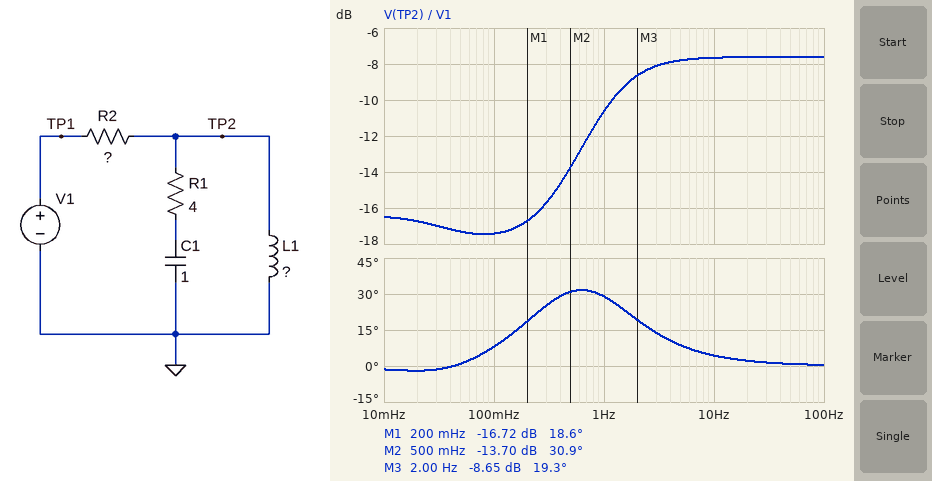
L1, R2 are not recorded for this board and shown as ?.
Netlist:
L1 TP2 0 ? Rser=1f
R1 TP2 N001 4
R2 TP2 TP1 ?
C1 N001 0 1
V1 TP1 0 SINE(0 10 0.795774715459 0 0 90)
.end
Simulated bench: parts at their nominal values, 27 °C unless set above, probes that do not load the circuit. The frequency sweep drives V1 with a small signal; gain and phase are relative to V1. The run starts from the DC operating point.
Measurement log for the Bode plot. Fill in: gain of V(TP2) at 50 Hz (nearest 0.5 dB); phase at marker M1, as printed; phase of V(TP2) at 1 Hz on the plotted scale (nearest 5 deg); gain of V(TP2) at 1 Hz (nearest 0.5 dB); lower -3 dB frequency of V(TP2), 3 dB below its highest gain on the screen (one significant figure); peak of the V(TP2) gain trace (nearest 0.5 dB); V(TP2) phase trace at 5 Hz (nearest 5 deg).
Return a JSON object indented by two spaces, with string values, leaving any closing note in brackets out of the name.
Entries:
{
  "gain of V(TP2) at 50 Hz": "-7.5 dB",
  "phase at marker M1, as printed": "18.6 deg",
  "phase of V(TP2) at 1 Hz on the plotted scale": "30 deg",
  "gain of V(TP2) at 1 Hz": "-10.5 dB",
  "lower -3 dB frequency of V(TP2), 3 dB below its highest gain on the screen": "1 Hz",
  "peak of the V(TP2) gain trace": "-7.5 dB",
  "V(TP2) phase trace at 5 Hz": "10 deg"
}
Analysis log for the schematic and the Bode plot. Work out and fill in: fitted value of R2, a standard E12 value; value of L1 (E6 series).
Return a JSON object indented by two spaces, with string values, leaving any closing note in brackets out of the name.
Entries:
{
  "fitted value of R2, a standard E12 value": "5.6 Ω",
  "value of L1": "470 mH"
}
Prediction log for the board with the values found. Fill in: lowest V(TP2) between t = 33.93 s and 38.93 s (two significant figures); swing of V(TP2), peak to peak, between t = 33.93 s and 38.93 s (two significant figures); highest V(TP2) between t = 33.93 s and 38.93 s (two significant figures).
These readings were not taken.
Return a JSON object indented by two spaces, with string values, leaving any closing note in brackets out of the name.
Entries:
{
  "lowest V(TP2) between t = 33.93 s and 38.93 s": "-2.6 V",
  "swing of V(TP2), peak to peak, between t = 33.93 s and 38.93 s": "5.3 V",
  "highest V(TP2) between t = 33.93 s and 38.93 s": "2.6 V"
}
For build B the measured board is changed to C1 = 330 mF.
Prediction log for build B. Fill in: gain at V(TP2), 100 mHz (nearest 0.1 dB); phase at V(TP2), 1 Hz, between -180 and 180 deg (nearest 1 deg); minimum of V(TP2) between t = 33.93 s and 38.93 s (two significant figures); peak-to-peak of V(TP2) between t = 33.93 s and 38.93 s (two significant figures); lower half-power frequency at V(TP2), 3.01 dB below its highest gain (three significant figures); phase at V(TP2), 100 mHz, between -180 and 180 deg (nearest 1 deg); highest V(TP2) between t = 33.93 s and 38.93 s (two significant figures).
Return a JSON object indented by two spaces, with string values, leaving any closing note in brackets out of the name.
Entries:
{
  "gain at V(TP2), 100 mHz": "-16.6 dB",
  "phase at V(TP2), 1 Hz, between -180 and 180 deg": "27 deg",
  "minimum of V(TP2) between t = 33.93 s and 38.93 s": "-2.7 V",
  "peak-to-peak of V(TP2) between t = 33.93 s and 38.93 s": "5.4 V",
  "lower half-power frequency at V(TP2), 3.01 dB below its highest gain": "958 mHz",
  "phase at V(TP2), 100 mHz, between -180 and 180 deg": "7 deg",
  "highest V(TP2) between t = 33.93 s and 38.93 s": "2.7 V"
}
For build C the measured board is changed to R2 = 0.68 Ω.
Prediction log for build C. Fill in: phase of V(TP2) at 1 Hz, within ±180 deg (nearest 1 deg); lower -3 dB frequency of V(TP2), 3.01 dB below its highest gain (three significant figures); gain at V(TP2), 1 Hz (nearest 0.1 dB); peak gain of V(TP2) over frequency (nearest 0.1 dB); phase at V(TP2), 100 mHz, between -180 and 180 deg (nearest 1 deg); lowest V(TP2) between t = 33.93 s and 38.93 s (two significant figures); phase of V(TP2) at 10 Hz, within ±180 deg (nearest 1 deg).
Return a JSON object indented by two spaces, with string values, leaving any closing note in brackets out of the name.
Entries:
{
  "phase of V(TP2) at 1 Hz, within ±180 deg": "9 deg",
  "lower -3 dB frequency of V(TP2), 3.01 dB below its highest gain": "231 mHz",
  "gain at V(TP2), 1 Hz": "-2.0 dB",
  "peak gain of V(TP2) over frequency": "-1.4 dB",
  "phase at V(TP2), 100 mHz, between -180 and 180 deg": "4 deg",
  "lowest V(TP2) between t = 33.93 s and 38.93 s": "-7.7 V",
  "phase of V(TP2) at 10 Hz, within ±180 deg": "1 deg"
}
